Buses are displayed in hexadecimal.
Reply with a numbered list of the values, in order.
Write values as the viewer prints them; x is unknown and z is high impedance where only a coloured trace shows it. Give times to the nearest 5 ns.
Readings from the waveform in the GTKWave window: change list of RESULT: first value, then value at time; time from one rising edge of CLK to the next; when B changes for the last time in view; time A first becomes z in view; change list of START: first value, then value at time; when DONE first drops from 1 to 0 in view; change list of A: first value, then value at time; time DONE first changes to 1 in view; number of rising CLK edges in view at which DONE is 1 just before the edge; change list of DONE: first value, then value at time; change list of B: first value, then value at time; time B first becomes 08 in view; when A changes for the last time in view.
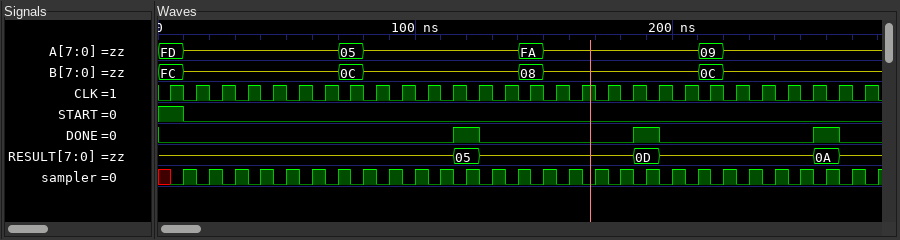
1. z, 05 at 115 ns, z at 125 ns, 0D at 185 ns, z at 195 ns, 0A at 255 ns, z at 265 ns
2. 10 ns
3. 220 ns
4. 10 ns
5. 1, 0 at 10 ns
6. 125 ns
7. FD, z at 10 ns, 05 at 70 ns, z at 80 ns, FA at 140 ns, z at 150 ns, 09 at 210 ns, z at 220 ns
8. 115 ns
9. 3
10. 0, 1 at 115 ns, 0 at 125 ns, 1 at 185 ns, 0 at 195 ns, 1 at 255 ns, 0 at 265 ns
11. FC, z at 10 ns, 0C at 70 ns, z at 80 ns, 08 at 140 ns, z at 150 ns, 0C at 210 ns, z at 220 ns
12. 140 ns
13. 220 ns
